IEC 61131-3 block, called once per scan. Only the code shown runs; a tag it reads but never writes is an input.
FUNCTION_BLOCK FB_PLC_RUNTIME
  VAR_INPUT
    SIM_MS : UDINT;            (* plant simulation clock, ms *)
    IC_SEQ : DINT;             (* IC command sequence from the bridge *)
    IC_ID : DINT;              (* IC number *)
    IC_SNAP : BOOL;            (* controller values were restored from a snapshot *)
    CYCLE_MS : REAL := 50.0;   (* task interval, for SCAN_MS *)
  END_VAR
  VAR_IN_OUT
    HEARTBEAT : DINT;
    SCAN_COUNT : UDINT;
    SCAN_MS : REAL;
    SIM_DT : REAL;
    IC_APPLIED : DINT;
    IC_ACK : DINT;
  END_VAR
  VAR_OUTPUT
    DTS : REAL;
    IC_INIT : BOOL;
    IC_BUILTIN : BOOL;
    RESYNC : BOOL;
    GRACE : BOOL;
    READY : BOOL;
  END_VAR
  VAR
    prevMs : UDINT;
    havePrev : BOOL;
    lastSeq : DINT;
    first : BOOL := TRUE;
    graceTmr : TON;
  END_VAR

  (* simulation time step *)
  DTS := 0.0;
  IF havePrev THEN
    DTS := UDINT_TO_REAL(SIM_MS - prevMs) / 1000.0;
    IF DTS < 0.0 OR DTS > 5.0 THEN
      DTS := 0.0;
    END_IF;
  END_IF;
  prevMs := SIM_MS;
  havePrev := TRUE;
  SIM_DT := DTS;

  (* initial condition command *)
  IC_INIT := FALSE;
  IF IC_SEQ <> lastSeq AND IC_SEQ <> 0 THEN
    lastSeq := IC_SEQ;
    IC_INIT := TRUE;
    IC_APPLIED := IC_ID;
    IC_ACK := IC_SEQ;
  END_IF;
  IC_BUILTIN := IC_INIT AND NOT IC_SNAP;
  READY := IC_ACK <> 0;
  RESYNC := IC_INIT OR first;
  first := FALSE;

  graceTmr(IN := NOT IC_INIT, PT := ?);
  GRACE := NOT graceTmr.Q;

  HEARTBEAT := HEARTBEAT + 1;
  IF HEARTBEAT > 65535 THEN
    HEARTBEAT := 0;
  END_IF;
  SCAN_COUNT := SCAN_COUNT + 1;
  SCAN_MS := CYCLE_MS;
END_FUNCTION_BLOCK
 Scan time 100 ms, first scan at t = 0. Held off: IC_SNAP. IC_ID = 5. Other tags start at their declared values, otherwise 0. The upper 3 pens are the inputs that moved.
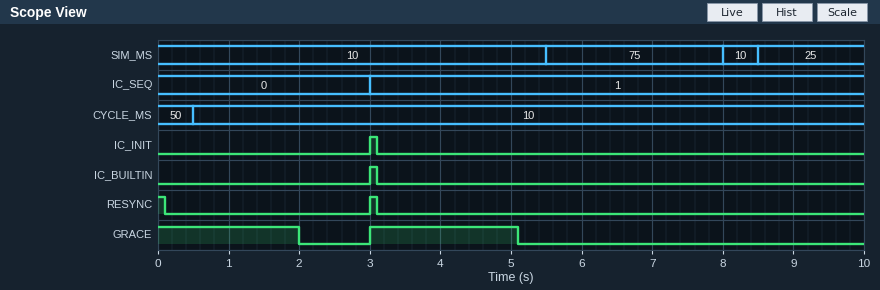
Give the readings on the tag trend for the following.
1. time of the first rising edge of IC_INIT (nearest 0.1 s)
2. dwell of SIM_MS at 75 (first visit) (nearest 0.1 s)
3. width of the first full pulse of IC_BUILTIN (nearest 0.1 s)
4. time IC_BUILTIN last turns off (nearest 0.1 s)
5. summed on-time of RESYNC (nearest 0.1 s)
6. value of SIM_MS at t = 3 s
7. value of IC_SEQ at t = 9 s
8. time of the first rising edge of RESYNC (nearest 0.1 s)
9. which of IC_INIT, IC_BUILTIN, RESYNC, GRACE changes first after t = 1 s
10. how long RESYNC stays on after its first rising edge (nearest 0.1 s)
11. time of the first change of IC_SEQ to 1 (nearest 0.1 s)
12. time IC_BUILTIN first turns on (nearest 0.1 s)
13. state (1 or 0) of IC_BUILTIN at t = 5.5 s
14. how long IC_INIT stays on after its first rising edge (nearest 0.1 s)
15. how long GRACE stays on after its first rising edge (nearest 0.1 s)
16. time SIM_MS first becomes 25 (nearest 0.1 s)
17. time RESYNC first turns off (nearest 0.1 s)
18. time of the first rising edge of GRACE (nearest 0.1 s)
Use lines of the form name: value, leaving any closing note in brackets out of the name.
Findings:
time of the first rising edge of IC_INIT: 3.0 s
dwell of SIM_MS at 75 (first visit): 2.5 s
width of the first full pulse of IC_BUILTIN: 0.1 s
time IC_BUILTIN last turns off: 3.1 s
summed on-time of RESYNC: 0.2 s
value of SIM_MS at t = 3 s: 10
value of IC_SEQ at t = 9 s: 1
time of the first rising edge of RESYNC: 3.0 s
which of IC_INIT, IC_BUILTIN, RESYNC, GRACE changes first after t = 1 s: GRACE
how long RESYNC stays on after its first rising edge: 0.1 s
time of the first change of IC_SEQ to 1: 3.0 s
time IC_BUILTIN first turns on: 3.0 s
state (1 or 0) of IC_BUILTIN at t = 5.5 s: 0
how long IC_INIT stays on after its first rising edge: 0.1 s
how long GRACE stays on after its first rising edge: 2.1 s
time SIM_MS first becomes 25: 8.5 s
time RESYNC first turns off: 0.1 s
time of the first rising edge of GRACE: 3.0 s
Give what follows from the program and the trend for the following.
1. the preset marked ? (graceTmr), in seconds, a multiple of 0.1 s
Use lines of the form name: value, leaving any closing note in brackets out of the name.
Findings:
the preset marked ? (graceTmr), in seconds, a multiple of 0.1 s: 2.0 s
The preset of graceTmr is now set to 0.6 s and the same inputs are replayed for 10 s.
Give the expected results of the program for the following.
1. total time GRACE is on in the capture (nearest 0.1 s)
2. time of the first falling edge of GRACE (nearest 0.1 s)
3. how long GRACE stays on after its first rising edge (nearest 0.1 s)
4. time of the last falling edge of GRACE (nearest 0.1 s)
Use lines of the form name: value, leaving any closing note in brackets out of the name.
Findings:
total time GRACE is on in the capture: 1.3 s
time of the first falling edge of GRACE: 0.6 s
how long GRACE stays on after its first rising edge: 0.7 s
time of the last falling edge of GRACE: 3.7 s
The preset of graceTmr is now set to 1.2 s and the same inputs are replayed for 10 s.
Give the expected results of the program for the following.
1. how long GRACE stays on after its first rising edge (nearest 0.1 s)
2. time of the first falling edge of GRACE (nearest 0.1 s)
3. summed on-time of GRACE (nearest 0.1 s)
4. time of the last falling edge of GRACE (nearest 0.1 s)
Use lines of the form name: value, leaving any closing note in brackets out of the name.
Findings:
how long GRACE stays on after its first rising edge: 1.3 s
time of the first falling edge of GRACE: 1.2 s
summed on-time of GRACE: 2.5 s
time of the last falling edge of GRACE: 4.3 s
